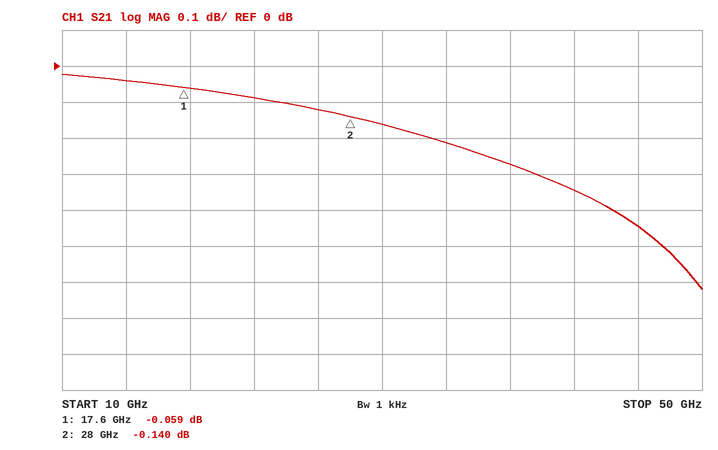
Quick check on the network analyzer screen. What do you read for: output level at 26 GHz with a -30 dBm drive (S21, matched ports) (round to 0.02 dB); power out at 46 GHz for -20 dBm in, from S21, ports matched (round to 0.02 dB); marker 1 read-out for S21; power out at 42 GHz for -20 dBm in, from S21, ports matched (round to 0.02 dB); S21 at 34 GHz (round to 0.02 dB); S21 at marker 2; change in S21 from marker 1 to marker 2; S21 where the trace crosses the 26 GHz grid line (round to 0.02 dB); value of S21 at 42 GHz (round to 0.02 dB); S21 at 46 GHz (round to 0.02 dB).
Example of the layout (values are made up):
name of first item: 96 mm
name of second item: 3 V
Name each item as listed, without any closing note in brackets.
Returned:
output level at 26 GHz with a -30 dBm drive (S21, matched ports): -30.12 dBm
power out at 46 GHz for -20 dBm in, from S21, ports matched: -20.44 dBm
marker 1 read-out for S21: -0.059 dB
power out at 42 GHz for -20 dBm in, from S21, ports matched: -20.34 dBm
S21 at 34 GHz: -0.22 dB
S21 at marker 2: -0.140 dB
change in S21 from marker 1 to marker 2: -0.081 dB
S21 where the trace crosses the 26 GHz grid line: -0.12 dB
value of S21 at 42 GHz: -0.34 dB
S21 at 46 GHz: -0.44 dB
